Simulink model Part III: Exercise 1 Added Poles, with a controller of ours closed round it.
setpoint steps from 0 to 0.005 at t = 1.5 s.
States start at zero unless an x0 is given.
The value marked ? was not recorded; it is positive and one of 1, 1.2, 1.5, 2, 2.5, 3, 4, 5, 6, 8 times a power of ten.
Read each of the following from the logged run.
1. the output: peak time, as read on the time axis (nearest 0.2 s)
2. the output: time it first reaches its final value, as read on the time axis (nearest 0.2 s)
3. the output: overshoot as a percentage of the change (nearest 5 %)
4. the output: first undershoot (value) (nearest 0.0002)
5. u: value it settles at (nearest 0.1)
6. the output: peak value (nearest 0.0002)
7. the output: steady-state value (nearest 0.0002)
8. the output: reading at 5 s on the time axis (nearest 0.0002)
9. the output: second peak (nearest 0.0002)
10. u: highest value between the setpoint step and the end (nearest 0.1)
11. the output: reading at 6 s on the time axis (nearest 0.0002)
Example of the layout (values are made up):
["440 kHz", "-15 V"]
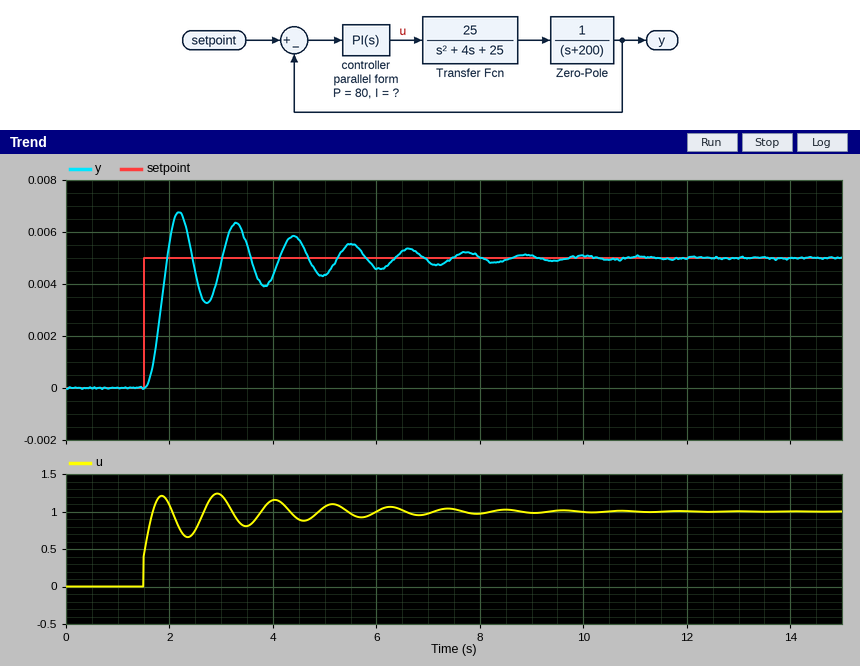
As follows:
["2.2 s", "2.0 s", "35 %", "0.0032", "1.0", "0.0068", "0.0050", "0.0044", "0.0064", "1.2", "0.0046"]
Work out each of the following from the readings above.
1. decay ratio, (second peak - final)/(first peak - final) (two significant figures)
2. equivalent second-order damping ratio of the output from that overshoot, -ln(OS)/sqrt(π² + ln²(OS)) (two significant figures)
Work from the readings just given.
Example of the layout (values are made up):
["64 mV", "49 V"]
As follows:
["0.78", "0.32"]
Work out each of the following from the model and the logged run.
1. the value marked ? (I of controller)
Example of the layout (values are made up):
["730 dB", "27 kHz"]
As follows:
["800"]
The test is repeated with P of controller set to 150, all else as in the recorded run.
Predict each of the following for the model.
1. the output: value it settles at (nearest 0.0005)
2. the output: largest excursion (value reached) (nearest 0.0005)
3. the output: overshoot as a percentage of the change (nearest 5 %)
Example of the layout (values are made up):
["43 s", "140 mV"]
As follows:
["0.0050", "0.0065", "25 %"]
